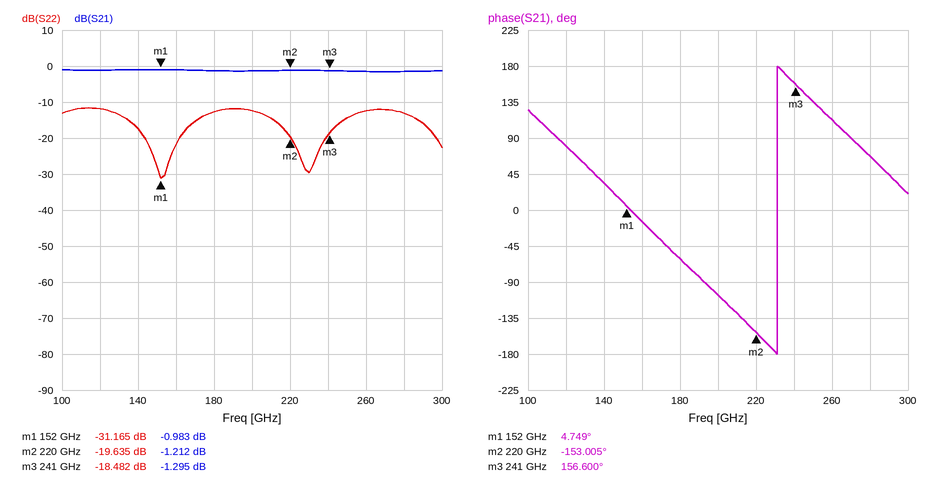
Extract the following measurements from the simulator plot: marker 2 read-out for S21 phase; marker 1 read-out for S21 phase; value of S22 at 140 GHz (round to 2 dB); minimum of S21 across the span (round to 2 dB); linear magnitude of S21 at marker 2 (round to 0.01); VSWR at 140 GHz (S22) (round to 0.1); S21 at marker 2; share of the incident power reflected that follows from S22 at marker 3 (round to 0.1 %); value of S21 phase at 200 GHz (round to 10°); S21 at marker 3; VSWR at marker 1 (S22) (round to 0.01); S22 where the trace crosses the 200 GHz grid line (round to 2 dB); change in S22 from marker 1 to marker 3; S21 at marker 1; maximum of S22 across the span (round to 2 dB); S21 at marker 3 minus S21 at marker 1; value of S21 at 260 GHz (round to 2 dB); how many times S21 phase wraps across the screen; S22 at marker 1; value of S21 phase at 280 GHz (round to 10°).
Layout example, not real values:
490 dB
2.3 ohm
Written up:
-153.005°
4.749°
-18 dB
-2 dB
0.87
1.3
-1.212 dB
1.4 %
-110°
-1.295 dB
1.06
-12 dB
12.683 dB
-0.983 dB
-12 dB
-0.312 dB
-2 dB
1
-31.165 dB
70°
